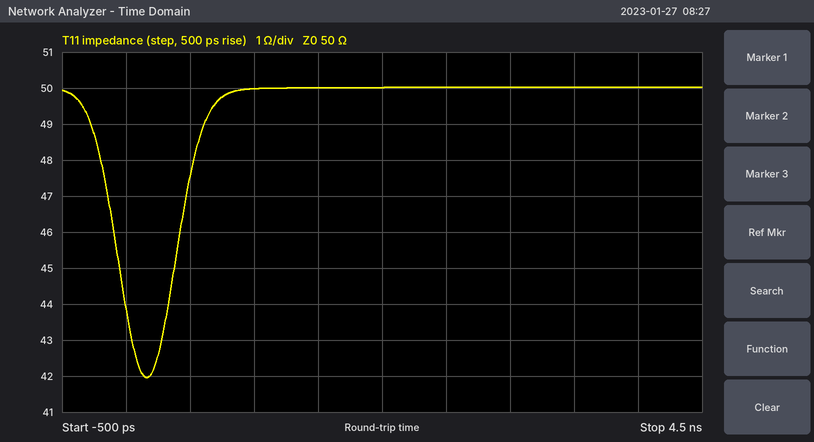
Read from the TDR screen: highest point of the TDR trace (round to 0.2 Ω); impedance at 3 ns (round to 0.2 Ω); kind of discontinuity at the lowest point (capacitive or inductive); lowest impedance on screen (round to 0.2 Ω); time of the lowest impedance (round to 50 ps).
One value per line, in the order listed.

50.0 Ω
50.0 Ω
capacitive
42.0 Ω
150 ps
